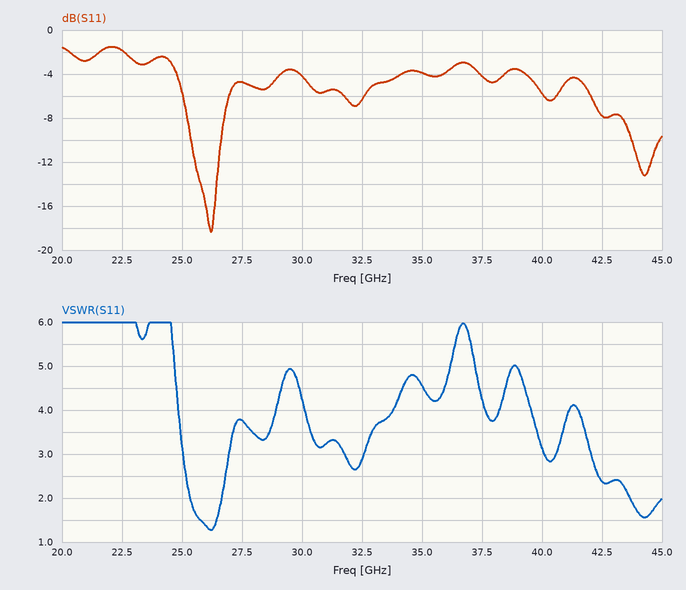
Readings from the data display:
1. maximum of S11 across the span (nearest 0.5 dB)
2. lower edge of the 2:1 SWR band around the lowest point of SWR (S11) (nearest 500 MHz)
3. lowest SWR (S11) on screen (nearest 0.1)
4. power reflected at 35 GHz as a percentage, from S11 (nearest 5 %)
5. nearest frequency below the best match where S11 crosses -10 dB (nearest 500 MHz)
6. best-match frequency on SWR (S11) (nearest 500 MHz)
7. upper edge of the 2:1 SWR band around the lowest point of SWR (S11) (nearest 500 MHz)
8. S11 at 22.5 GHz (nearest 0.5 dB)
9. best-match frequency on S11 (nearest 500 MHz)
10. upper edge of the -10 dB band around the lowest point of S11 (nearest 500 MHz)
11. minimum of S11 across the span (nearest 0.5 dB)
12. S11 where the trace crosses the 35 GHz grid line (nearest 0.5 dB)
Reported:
-1.5 dB
25.5 GHz
1.3
40 %
25.5 GHz
26.0 GHz
26.5 GHz
-2.0 dB
26.0 GHz
26.5 GHz
-18.5 dB
-4.0 dB
